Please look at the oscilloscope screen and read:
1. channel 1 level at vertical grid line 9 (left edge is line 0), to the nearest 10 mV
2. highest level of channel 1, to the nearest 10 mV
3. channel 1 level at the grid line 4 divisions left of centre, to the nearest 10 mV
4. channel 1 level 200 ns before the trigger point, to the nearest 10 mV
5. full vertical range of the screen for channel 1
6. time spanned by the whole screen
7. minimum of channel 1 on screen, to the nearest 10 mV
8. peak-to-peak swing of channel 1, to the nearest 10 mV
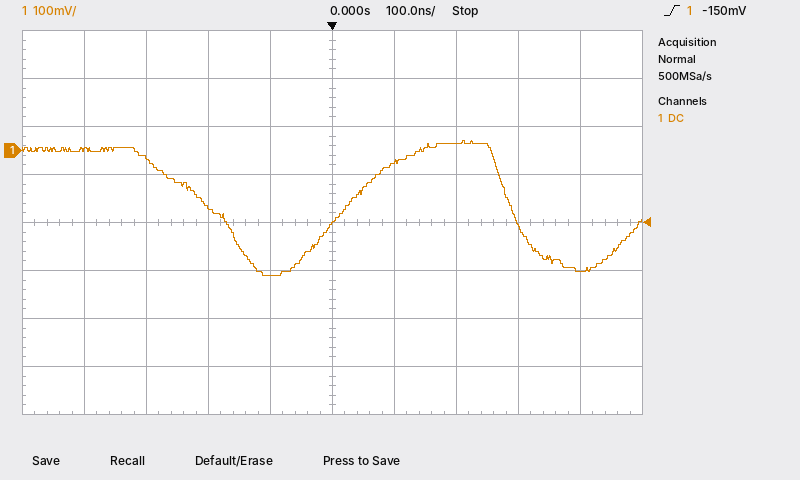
-250 mV
20 mV
0 mV
-120 mV
800 mV
1 µs
-260 mV
280 mV
